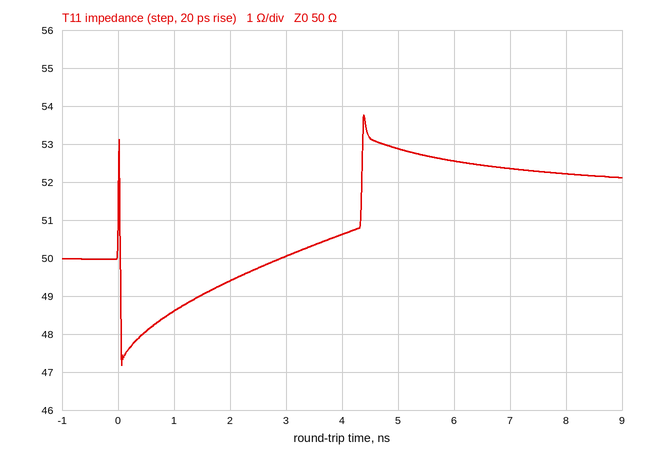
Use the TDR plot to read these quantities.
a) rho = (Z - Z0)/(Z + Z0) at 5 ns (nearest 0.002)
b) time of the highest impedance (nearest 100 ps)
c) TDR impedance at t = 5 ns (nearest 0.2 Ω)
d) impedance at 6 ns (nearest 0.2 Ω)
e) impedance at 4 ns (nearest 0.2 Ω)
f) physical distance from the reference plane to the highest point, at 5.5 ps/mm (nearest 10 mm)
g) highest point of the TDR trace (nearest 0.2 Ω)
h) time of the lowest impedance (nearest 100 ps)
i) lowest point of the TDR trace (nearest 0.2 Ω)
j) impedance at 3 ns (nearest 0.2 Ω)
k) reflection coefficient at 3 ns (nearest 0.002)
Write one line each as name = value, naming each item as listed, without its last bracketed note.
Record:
rho = (Z - Z0)/(Z + Z0) at 5 ns = +0.028
time of the highest impedance = 4.4 ns
TDR impedance at t = 5 ns = 52.8 Ω
impedance at 6 ns = 52.6 Ω
impedance at 4 ns = 50.6 Ω
physical distance from the reference plane to the highest point, at 5.5 ps/mm = 400 mm
highest point of the TDR trace = 53.8 Ω
time of the lowest impedance = 100 ps
lowest point of the TDR trace = 47.2 Ω
impedance at 3 ns = 50.0 Ω
reflection coefficient at 3 ns = 0.000
